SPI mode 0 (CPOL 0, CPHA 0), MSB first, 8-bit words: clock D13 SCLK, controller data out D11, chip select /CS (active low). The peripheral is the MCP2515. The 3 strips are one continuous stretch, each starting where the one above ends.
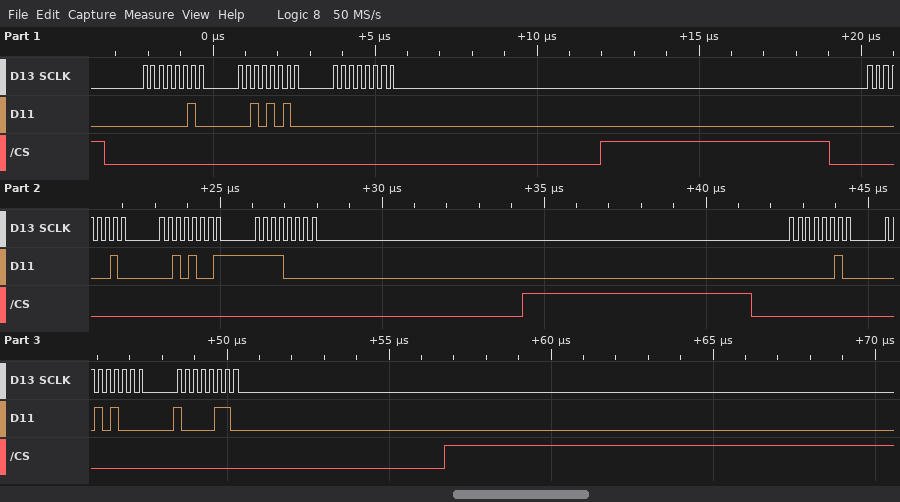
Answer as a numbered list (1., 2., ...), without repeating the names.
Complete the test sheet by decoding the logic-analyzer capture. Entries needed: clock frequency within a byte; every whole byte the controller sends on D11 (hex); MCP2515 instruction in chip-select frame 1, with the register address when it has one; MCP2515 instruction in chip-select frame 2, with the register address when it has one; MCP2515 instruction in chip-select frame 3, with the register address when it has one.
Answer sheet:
1. 4 MHz
2. 0x02 0x2A 0x00 0x02 0x29 0xF0 0x02 0x28 0x86
3. WRITE 0x2A
4. WRITE 0x29
5. WRITE 0x28
